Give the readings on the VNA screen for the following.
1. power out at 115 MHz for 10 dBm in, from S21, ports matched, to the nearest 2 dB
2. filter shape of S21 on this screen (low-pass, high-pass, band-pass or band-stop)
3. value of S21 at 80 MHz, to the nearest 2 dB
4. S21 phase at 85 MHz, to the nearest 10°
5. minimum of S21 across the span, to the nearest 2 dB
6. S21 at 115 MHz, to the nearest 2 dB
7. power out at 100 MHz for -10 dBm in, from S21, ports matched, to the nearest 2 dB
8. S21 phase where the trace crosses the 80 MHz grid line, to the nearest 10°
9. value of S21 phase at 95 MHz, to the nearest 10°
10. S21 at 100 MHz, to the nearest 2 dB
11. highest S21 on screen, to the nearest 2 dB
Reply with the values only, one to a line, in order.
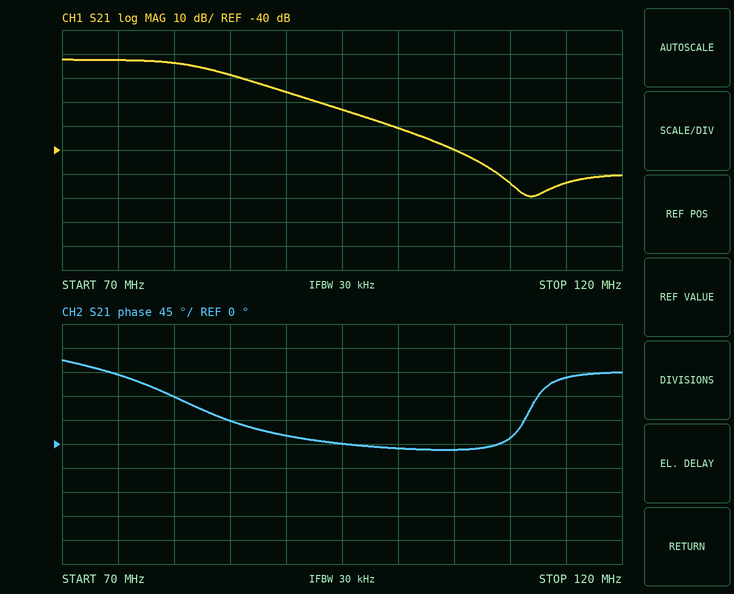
-44 dBm
low-pass
-4 dB
40°
-60 dB
-54 dB
-40 dBm
90°
0°
-30 dB
-2 dB
